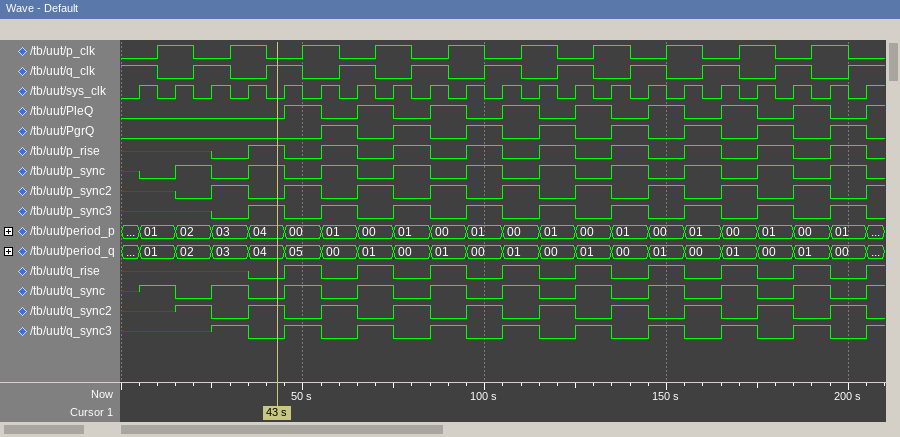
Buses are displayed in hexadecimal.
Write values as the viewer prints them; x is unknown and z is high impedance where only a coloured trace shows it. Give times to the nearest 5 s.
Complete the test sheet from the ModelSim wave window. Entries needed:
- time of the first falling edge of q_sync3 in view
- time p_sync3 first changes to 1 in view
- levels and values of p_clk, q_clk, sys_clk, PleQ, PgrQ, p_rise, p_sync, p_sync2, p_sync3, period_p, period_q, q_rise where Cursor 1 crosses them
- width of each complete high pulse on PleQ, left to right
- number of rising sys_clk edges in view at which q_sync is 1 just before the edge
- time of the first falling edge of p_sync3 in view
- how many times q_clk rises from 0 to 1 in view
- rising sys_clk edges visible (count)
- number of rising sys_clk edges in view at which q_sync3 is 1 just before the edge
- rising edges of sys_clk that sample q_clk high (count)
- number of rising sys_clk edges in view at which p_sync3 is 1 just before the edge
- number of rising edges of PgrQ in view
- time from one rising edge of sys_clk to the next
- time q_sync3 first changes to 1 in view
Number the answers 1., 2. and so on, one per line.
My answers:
1. 35 s
2. 35 s
3. p_clk=0, q_clk=1, sys_clk=0, PleQ=0, PgrQ=0, p_rise=1, p_sync=1, p_sync2=0, p_sync3=1, period_p=04, period_q=04, q_rise=0
4. 10 s, 10 s, 10 s, 10 s, 10 s, 10 s, 10 s, 10 s
5. 10
6. 45 s
7. 10
8. 21
9. 9
10. 11
11. 9
12. 8
13. 10 s
14. 25 s
